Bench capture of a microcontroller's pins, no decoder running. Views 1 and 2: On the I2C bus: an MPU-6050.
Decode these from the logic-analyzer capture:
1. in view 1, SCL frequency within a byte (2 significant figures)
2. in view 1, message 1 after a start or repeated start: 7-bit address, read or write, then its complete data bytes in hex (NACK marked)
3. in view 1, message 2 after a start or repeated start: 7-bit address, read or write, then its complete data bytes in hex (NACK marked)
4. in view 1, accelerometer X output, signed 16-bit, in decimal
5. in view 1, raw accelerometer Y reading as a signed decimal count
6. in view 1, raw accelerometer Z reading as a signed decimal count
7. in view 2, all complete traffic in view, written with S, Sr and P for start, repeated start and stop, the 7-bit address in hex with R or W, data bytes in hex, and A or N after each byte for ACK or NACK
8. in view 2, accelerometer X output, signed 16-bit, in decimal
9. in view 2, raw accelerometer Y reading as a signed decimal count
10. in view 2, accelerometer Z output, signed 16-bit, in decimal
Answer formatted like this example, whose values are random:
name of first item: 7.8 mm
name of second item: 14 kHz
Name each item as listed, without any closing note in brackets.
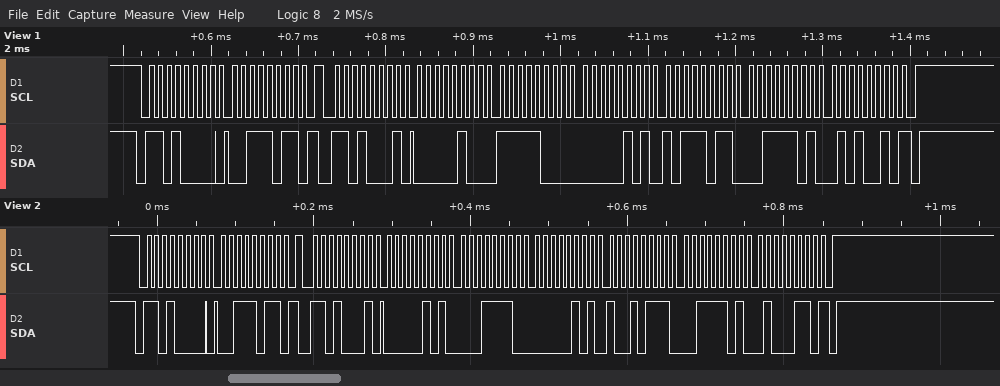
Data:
in view 1, SCL frequency within a byte: 100 kHz
in view 1, message 1 after a start or repeated start: 7-bit address, read or write, then its complete data bytes in hex: 0x68 write: 3B
in view 1, message 2 after a start or repeated start: 7-bit address, read or write, then its complete data bytes in hex: 0x68 read: 04 F8 05 BB 3D 52 NACK
in view 1, accelerometer X output, signed 16-bit, in decimal: 1272
in view 1, raw accelerometer Y reading as a signed decimal count: 1467
in view 1, raw accelerometer Z reading as a signed decimal count: 15698
in view 2, all complete traffic in view, written with S, Sr and P for start, repeated start and stop, the 7-bit address in hex with R or W, data bytes in hex, and A or N after each byte for ACK or NACK: S 68W A 3B A Sr 68R A 05 A 1E A 05 A 97 A 3D A 46 N P
in view 2, accelerometer X output, signed 16-bit, in decimal: 1310
in view 2, raw accelerometer Y reading as a signed decimal count: 1431
in view 2, accelerometer Z output, signed 16-bit, in decimal: 15686
